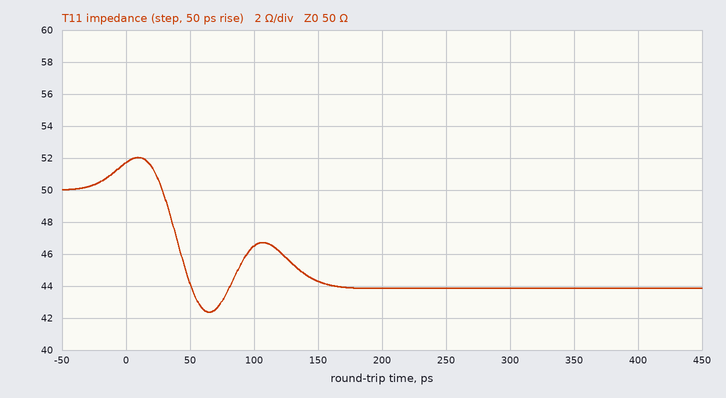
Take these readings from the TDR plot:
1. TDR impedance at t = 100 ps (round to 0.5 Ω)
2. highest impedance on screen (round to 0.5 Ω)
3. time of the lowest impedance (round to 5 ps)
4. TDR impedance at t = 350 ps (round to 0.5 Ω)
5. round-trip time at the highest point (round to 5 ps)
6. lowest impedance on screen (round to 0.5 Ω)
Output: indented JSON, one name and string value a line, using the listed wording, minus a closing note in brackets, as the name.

{
  "TDR impedance at t = 100 ps": "46.5 Ω",
  "highest impedance on screen": "52.0 Ω",
  "time of the lowest impedance": "65 ps",
  "TDR impedance at t = 350 ps": "44.0 Ω",
  "round-trip time at the highest point": "10 ps",
  "lowest impedance on screen": "42.5 Ω"
}
